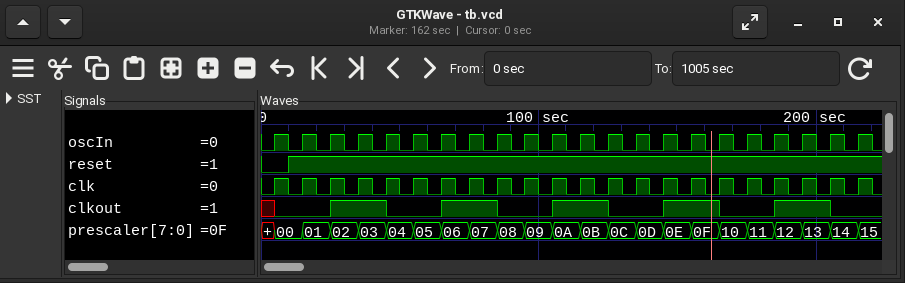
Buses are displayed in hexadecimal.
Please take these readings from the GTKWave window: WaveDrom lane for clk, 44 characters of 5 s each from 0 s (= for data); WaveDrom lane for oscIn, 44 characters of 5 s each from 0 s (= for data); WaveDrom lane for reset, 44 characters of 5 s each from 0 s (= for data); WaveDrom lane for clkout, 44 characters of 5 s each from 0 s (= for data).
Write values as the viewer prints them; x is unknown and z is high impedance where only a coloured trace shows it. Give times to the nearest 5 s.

{name: 'clk', wave: '01010101010101010101010101010101010101010101'}
{name: 'oscIn', wave: '01010101010101010101010101010101010101010101'}
{name: 'reset', wave: '0.1.........................................'}
{name: 'clkout', wave: 'x0...1...0...1...0...1...0...1...0...1...0..'}
